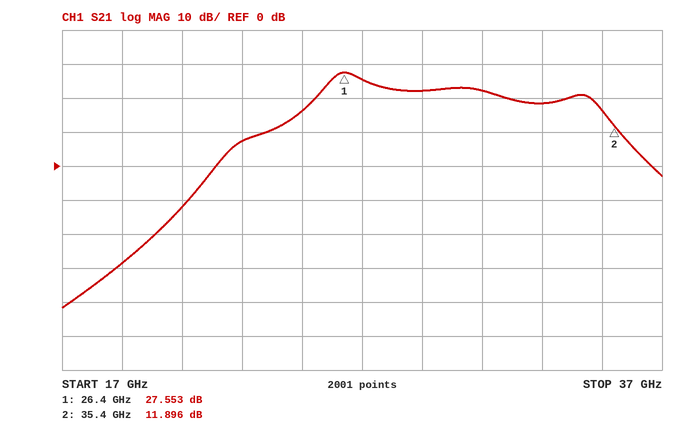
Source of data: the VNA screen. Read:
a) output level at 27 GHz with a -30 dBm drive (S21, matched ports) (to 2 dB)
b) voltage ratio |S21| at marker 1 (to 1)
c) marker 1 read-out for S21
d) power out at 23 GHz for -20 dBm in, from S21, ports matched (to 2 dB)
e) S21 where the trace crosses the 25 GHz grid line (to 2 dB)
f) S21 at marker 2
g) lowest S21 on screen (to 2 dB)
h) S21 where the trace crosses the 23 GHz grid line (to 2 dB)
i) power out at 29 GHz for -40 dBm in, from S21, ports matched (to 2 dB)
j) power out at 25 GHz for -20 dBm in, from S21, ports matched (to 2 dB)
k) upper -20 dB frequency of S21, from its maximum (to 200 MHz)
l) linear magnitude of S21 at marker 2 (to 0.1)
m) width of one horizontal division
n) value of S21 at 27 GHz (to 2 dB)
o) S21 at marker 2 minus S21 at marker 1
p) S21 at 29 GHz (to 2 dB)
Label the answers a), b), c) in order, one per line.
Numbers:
a) -4 dBm
b) 24
c) 27.553 dB
d) -12 dBm
e) 16 dB
f) 11.896 dB
g) -42 dB
h) 8 dB
i) -18 dBm
j) -4 dBm
k) 35.8 GHz
l) 3.9
m) 2 GHz
n) 26 dB
o) -15.657 dB
p) 22 dB
